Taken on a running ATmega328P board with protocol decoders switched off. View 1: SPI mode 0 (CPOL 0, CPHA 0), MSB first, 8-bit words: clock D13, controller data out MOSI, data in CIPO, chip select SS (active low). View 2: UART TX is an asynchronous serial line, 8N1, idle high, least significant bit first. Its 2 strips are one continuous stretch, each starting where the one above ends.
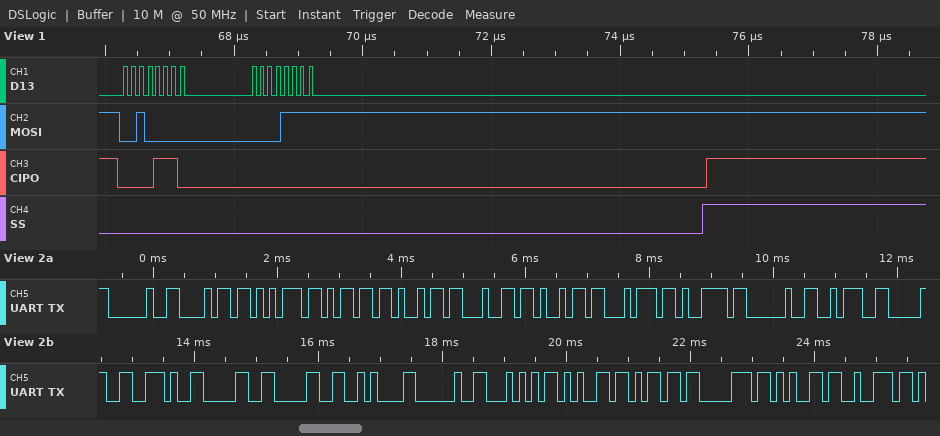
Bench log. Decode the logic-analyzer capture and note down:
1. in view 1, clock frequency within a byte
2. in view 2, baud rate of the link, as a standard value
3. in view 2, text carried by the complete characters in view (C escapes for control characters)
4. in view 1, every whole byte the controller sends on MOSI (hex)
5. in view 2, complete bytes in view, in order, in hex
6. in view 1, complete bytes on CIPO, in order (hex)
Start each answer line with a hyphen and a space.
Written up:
- 8 MHz
- 9600 baud
- " humidity :0.00\n Temper"
- 20 0F
- 20 68 75 6D 69 64 69 74 79 20 3A 30 2E 30 30 0A 20 54 65 6D 70 65 72
- 0E 00
